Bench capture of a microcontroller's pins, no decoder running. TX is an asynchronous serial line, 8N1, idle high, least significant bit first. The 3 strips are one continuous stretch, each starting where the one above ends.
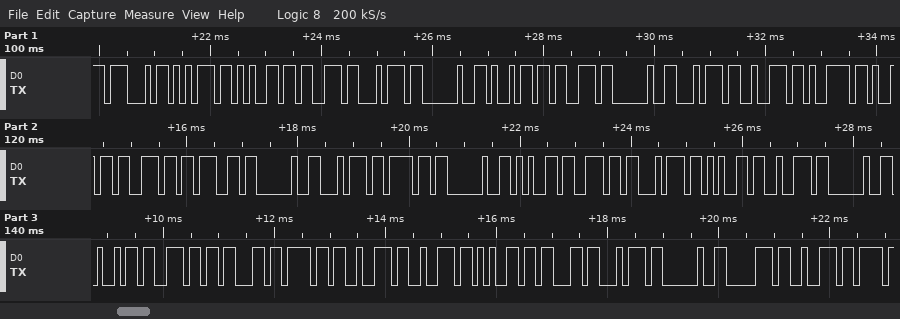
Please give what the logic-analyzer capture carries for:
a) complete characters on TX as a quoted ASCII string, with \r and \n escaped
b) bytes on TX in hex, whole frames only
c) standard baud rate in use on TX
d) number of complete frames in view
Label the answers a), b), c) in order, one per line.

a) "Guest is trying to enter incorrect pr"
b) 47 75 65 73 74 20 69 73 20 74 72 79 69 6E 67 20 74 6F 20 65 6E 74 65 72 20 69 6E 63 6F 72 72 65 63 74 20 70 72
c) 9600 baud
d) 37
